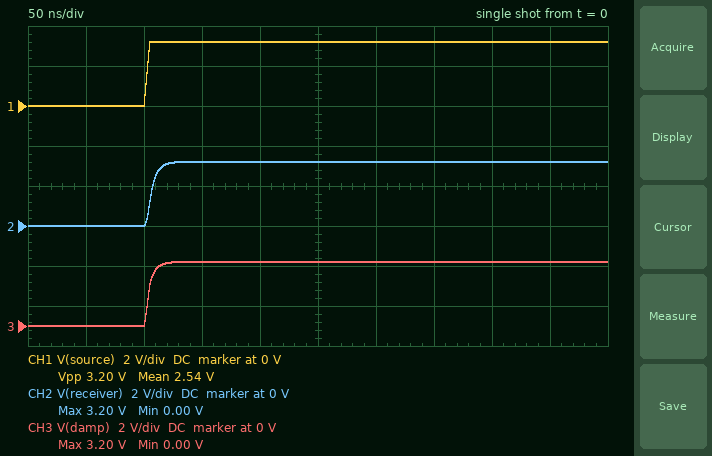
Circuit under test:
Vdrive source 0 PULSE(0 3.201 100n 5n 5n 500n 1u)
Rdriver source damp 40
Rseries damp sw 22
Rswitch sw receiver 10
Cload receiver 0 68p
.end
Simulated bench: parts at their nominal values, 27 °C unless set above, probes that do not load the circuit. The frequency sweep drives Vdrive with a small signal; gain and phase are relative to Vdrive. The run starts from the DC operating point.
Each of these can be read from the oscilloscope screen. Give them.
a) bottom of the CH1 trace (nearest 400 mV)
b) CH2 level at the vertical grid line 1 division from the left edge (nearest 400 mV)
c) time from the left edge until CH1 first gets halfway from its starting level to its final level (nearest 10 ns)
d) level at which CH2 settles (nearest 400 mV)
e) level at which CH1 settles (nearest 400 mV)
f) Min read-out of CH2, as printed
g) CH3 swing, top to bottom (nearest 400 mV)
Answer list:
0 V
0 V
100 ns
3.2 V
3.2 V
0.00 V
3.2 V
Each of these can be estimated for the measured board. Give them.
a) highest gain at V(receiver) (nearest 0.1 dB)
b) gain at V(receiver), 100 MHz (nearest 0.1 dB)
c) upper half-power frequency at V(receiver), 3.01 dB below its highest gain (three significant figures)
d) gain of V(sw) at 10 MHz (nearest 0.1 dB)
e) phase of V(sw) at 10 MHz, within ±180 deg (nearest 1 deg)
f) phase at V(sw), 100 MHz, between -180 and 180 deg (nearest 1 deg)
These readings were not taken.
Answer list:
0 dB
-10.2 dB
32.5 MHz
-0.4 dB
-15 deg
-49 deg
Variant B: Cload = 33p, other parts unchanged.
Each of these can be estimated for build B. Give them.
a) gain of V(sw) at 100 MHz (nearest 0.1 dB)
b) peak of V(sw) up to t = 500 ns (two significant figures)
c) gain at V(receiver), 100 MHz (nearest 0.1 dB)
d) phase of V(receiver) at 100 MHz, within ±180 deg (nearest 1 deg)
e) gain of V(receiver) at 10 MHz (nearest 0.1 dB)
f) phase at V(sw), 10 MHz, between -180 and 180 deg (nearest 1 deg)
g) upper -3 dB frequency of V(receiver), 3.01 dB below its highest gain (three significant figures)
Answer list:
-4.9 dB
3.2 V
-5.1 dB
-56 deg
-0.1 dB
-7 deg
67.0 MHz
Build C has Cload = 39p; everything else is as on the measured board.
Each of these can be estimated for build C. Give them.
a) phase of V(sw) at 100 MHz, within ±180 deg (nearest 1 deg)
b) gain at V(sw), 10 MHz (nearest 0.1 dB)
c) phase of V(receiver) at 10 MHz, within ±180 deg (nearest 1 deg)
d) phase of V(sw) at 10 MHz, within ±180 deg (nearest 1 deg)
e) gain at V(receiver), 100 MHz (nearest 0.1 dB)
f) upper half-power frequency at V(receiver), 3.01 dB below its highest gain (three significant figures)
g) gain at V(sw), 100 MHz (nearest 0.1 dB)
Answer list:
-47 deg
-0.1 dB
-10 deg
-9 deg
-6.1 dB
56.7 MHz
-5.9 dB
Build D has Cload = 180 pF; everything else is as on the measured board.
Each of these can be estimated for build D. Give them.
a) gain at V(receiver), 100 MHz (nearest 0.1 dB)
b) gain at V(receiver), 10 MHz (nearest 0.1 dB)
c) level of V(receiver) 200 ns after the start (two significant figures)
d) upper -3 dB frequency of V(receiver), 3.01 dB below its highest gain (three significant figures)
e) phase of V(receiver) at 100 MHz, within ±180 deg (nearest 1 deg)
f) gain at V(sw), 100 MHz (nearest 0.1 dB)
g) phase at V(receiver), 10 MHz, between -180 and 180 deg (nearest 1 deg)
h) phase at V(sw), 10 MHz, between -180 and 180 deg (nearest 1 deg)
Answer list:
-18.3 dB
-2.2 dB
3.2 V
12.3 MHz
-83 deg
-14.7 dB
-39 deg
-33 deg
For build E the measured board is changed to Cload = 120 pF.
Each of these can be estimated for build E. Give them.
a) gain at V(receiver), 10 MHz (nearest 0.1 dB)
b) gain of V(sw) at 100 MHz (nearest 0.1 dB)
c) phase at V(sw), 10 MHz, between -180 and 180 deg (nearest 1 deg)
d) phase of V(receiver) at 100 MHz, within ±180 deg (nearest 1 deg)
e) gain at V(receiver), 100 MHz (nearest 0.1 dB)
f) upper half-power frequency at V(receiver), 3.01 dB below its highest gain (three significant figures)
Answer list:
-1.1 dB
-12.9 dB
-24 deg
-80 deg
-14.8 dB
18.4 MHz
